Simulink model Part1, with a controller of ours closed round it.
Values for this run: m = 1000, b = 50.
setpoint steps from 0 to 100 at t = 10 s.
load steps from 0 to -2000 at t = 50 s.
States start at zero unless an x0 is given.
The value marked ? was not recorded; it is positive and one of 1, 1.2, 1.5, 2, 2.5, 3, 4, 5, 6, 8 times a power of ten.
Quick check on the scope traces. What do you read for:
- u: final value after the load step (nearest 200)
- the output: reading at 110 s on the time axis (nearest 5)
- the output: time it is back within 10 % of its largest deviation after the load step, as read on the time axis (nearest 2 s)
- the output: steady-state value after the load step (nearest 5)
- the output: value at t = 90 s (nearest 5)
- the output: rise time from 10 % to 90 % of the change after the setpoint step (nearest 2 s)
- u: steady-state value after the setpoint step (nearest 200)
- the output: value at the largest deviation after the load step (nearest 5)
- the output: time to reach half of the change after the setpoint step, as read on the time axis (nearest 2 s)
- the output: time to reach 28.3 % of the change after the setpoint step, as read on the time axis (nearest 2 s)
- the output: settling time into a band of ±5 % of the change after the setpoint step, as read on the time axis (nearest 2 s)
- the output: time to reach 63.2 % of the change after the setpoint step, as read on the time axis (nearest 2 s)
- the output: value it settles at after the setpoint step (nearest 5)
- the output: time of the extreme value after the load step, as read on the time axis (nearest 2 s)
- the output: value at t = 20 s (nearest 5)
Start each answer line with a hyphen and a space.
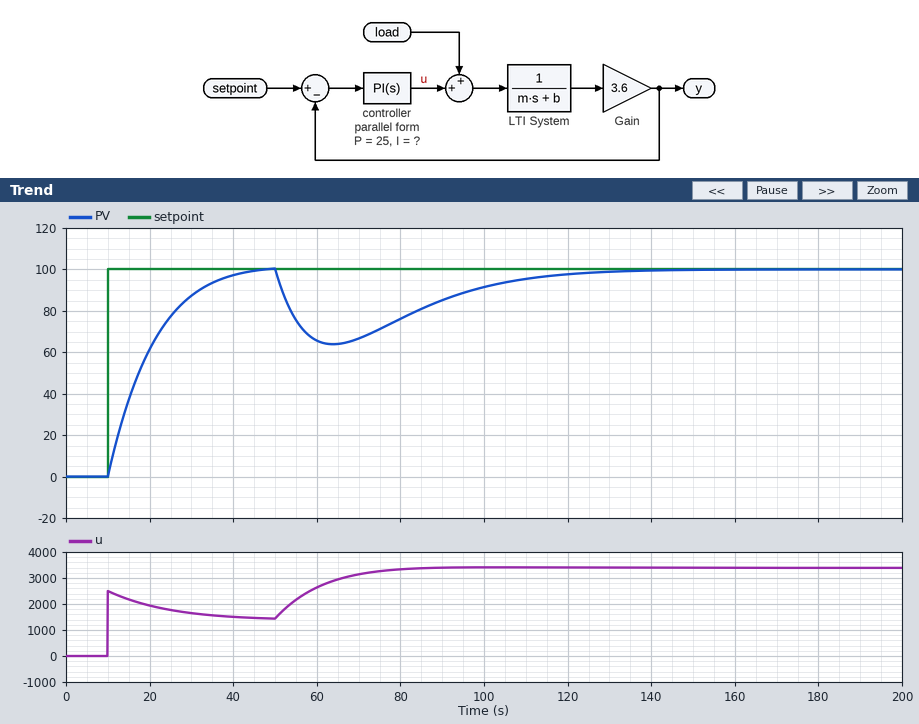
- 3400
- 95
- 114 s
- 100
- 85
- 20 s
- 1400
- 65
- 18 s
- 14 s
- 36 s
- 20 s
- 100
- 64 s
- 60
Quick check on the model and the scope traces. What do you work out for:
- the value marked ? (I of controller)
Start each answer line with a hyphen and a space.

- 1.5
